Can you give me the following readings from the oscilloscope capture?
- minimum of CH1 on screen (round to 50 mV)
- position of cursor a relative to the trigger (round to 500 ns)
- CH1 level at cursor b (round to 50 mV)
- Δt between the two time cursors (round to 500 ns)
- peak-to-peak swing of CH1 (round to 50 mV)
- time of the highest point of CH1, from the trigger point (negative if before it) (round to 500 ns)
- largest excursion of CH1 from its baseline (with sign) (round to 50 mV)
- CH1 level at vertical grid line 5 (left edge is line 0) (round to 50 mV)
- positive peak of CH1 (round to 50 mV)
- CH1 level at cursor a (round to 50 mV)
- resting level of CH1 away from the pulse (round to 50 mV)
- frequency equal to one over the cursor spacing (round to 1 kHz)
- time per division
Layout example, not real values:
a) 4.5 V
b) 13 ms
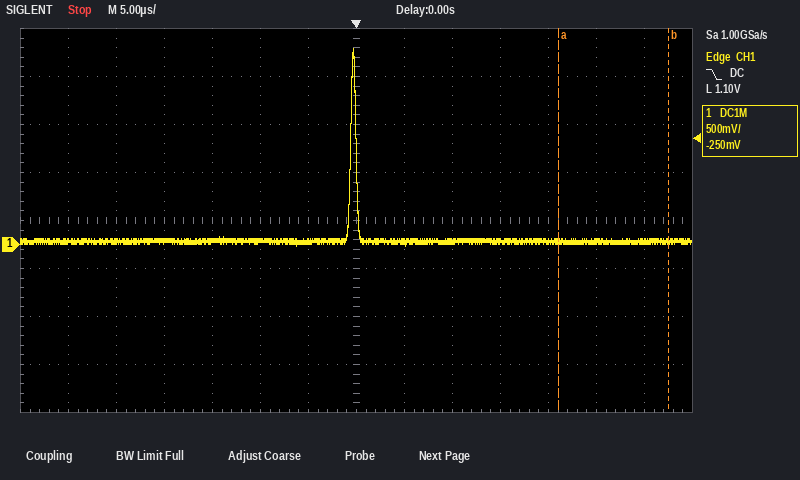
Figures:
a) 0 mV
b) +21.0 µs
c) 50 mV
d) 11.5 µs
e) 2.05 V
f) -500 ns
g) +2.00 V
h) 50 mV
i) 2.05 V
j) 50 mV
k) 50 mV
l) 87 kHz
m) 5 µs
